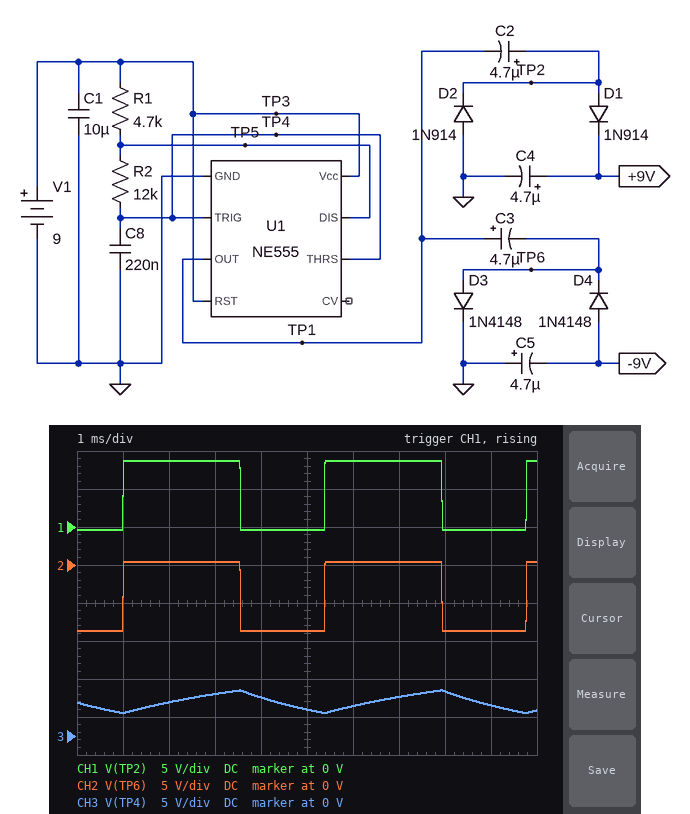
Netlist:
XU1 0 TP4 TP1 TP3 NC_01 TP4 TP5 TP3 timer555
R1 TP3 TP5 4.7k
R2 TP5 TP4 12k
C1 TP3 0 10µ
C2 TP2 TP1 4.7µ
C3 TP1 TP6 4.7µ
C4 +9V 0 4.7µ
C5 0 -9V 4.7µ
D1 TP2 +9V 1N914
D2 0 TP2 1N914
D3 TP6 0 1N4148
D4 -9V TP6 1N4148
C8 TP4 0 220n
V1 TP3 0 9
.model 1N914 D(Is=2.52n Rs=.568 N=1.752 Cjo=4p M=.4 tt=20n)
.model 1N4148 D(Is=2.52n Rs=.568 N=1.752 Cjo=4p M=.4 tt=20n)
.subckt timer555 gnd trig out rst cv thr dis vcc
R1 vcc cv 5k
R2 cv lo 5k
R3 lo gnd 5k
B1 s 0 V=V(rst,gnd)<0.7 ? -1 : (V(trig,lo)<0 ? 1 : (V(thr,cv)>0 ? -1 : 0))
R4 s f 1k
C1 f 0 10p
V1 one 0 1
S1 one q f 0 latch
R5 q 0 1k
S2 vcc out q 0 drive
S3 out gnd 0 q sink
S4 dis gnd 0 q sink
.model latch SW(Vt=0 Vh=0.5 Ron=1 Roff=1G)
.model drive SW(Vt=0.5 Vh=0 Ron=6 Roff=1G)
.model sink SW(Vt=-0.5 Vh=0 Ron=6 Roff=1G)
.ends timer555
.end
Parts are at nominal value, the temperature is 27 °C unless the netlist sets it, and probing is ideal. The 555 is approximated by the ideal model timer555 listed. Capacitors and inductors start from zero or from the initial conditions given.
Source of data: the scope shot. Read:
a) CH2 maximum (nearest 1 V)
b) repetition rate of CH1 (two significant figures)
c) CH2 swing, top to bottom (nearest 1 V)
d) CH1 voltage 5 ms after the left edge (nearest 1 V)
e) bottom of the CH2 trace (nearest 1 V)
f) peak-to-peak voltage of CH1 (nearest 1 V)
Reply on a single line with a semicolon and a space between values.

0 V; 230 Hz; 9 V; 0 V; -9 V; 9 V
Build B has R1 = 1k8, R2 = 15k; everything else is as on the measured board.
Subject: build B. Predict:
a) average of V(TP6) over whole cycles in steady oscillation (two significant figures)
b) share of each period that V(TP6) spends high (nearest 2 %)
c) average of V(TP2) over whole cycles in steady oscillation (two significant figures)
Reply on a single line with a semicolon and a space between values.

-3.9 V; 52 %; 4.4 V
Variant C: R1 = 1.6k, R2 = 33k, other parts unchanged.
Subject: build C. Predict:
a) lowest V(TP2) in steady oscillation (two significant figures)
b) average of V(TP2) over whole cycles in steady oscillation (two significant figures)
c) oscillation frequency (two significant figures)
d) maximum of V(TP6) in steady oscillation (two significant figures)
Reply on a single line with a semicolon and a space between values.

-360 mV; 4.2 V; 97 Hz; 360 mV
